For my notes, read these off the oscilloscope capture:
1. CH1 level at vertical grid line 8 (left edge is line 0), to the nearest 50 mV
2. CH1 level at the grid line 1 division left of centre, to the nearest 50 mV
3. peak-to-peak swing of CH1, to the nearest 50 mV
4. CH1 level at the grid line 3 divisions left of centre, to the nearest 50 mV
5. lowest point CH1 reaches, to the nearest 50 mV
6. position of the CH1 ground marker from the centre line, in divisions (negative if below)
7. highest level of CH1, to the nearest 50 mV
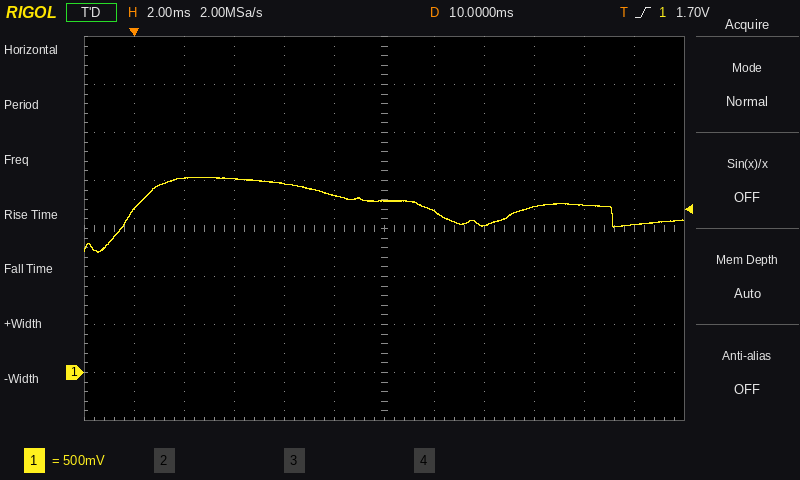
1.55 V
1.85 V
800 mV
2.00 V
1.25 V
-3.0 div
2.05 V
